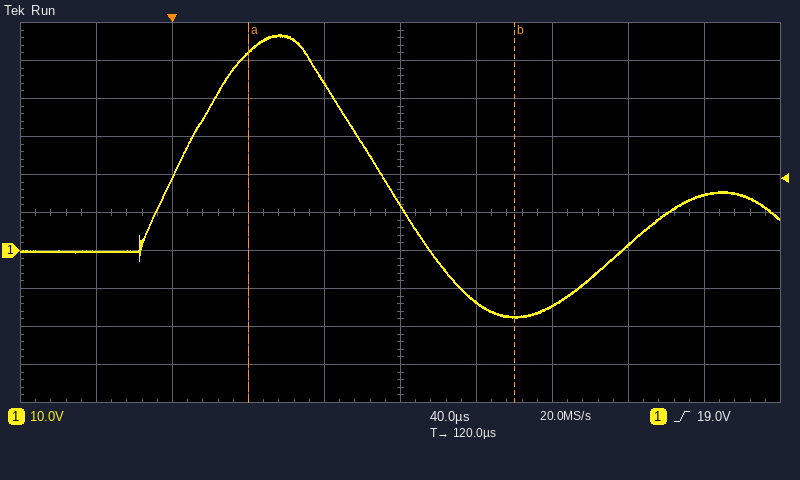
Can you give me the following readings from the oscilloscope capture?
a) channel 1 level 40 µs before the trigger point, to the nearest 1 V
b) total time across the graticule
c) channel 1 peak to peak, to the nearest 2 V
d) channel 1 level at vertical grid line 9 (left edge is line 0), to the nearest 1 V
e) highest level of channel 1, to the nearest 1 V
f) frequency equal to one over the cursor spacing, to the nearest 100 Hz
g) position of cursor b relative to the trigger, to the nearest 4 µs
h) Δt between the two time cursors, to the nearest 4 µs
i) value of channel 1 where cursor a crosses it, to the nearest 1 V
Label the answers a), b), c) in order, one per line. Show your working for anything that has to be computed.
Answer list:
a) 0 V
b) 400 µs
c) 74 V
d) 15 V
e) 57 V
f) 1 / 140 µs ≈ 7.1 kHz
g) +180 µs
h) 140 µs
i) 52 V
